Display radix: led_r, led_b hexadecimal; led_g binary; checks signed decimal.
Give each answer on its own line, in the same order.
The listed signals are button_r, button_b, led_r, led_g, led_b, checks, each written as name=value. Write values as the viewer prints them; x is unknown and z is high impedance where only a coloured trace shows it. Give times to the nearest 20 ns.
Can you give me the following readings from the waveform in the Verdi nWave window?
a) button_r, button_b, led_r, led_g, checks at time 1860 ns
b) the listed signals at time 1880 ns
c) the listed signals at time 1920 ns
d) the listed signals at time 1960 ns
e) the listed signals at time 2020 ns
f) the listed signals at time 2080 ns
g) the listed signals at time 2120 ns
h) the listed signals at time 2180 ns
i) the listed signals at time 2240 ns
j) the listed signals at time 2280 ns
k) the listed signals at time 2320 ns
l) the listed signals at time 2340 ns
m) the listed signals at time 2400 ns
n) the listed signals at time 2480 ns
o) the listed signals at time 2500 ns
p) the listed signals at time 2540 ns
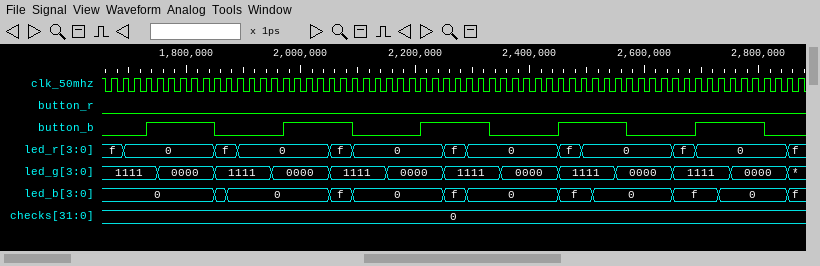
button_r=0, button_b=0, led_r=f, led_g=1111, checks=0
button_r=0, button_b=0, led_r=f, led_g=1111, led_b=0, checks=0
button_r=0, button_b=0, led_r=0, led_g=1111, led_b=0, checks=0
button_r=0, button_b=0, led_r=0, led_g=0000, led_b=0, checks=0
button_r=0, button_b=1, led_r=0, led_g=0000, led_b=0, checks=0
button_r=0, button_b=1, led_r=f, led_g=1111, led_b=f, checks=0
button_r=0, button_b=0, led_r=0, led_g=1111, led_b=0, checks=0
button_r=0, button_b=0, led_r=0, led_g=0000, led_b=0, checks=0
button_r=0, button_b=1, led_r=0, led_g=0000, led_b=0, checks=0
button_r=0, button_b=1, led_r=f, led_g=1111, led_b=f, checks=0
button_r=0, button_b=1, led_r=0, led_g=1111, led_b=0, checks=0
button_r=0, button_b=0, led_r=0, led_g=1111, led_b=0, checks=0
button_r=0, button_b=0, led_r=0, led_g=0000, led_b=0, checks=0
button_r=0, button_b=1, led_r=f, led_g=1111, led_b=f, checks=0
button_r=0, button_b=1, led_r=0, led_g=1111, led_b=f, checks=0
button_r=0, button_b=1, led_r=0, led_g=1111, led_b=0, checks=0
